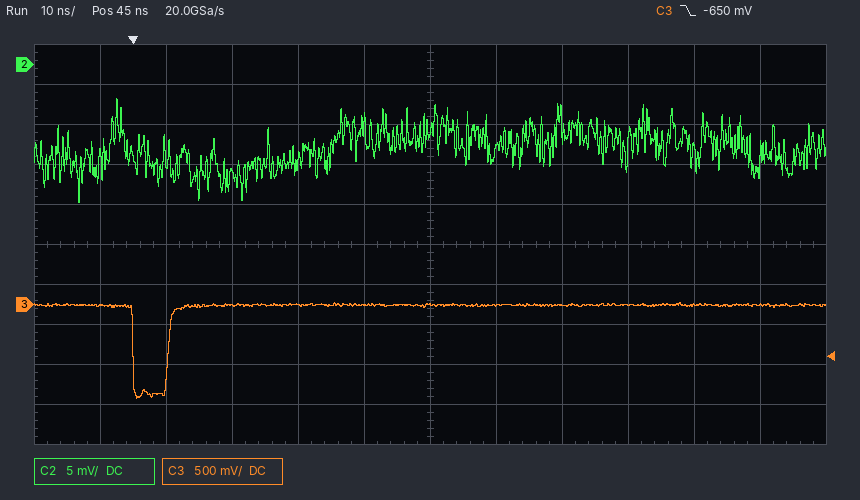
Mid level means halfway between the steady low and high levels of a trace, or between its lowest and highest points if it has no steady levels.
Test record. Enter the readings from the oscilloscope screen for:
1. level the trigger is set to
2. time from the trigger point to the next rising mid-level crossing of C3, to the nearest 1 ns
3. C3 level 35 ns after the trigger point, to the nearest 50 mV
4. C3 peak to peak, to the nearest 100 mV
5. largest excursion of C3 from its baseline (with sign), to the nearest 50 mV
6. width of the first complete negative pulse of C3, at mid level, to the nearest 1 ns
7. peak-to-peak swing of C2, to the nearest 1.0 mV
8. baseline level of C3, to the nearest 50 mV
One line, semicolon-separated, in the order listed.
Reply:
-650 mV; 5 ns; 0 mV; 1.20 V; -1.15 V; 5 ns; 13.0 mV; 0 mV
